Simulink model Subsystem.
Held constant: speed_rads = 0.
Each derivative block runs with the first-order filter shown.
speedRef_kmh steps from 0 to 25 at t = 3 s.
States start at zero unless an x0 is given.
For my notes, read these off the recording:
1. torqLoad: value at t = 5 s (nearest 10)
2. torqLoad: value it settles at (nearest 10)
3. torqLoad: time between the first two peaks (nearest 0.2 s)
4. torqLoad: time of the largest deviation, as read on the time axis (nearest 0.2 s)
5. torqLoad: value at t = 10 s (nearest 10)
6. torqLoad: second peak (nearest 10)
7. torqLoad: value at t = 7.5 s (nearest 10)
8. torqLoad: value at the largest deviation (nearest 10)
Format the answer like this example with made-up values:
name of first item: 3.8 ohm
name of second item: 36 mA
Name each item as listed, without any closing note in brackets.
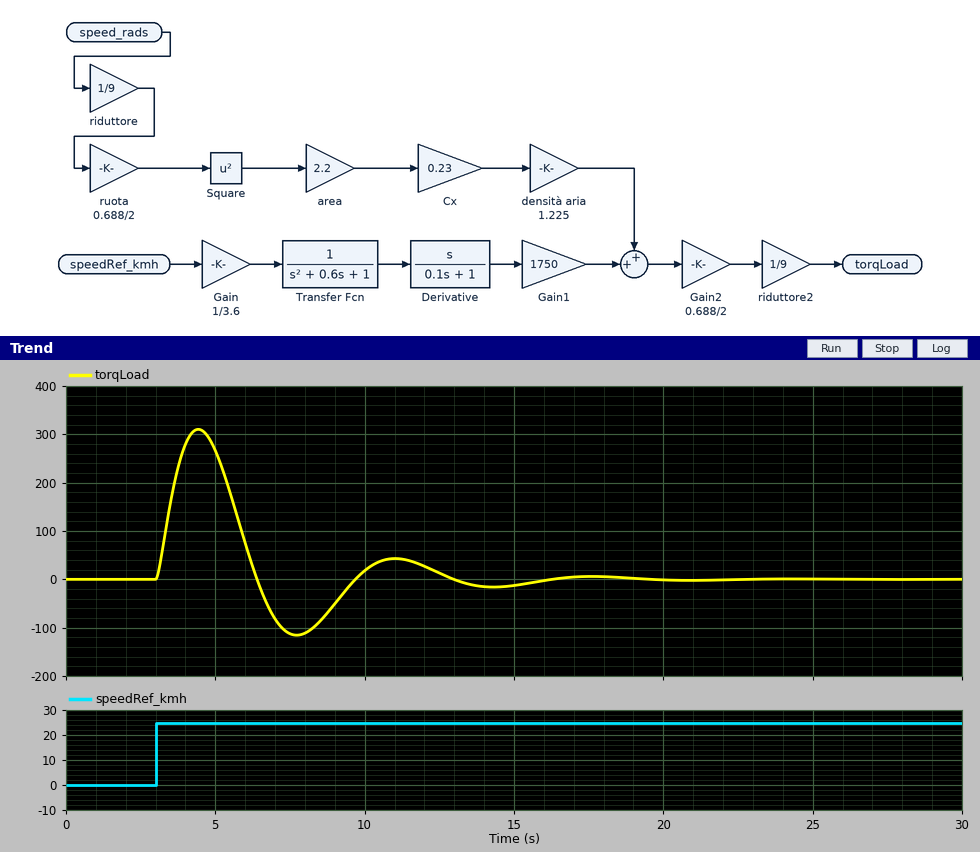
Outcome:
torqLoad: value at t = 5 s: 270
torqLoad: value it settles at: 0
torqLoad: time between the first two peaks: 6.6 s
torqLoad: time of the largest deviation, as read on the time axis: 4.4 s
torqLoad: value at t = 10 s: 20
torqLoad: second peak: 40
torqLoad: value at t = 7.5 s: -110
torqLoad: value at the largest deviation: 310
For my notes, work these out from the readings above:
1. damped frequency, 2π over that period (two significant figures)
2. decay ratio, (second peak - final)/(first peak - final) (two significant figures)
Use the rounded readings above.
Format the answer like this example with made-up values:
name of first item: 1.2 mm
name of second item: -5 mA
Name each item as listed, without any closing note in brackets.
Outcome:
damped frequency, 2π over that period: 0.95 rad/s
decay ratio, (second peak - final)/(first peak - final): 0.13
